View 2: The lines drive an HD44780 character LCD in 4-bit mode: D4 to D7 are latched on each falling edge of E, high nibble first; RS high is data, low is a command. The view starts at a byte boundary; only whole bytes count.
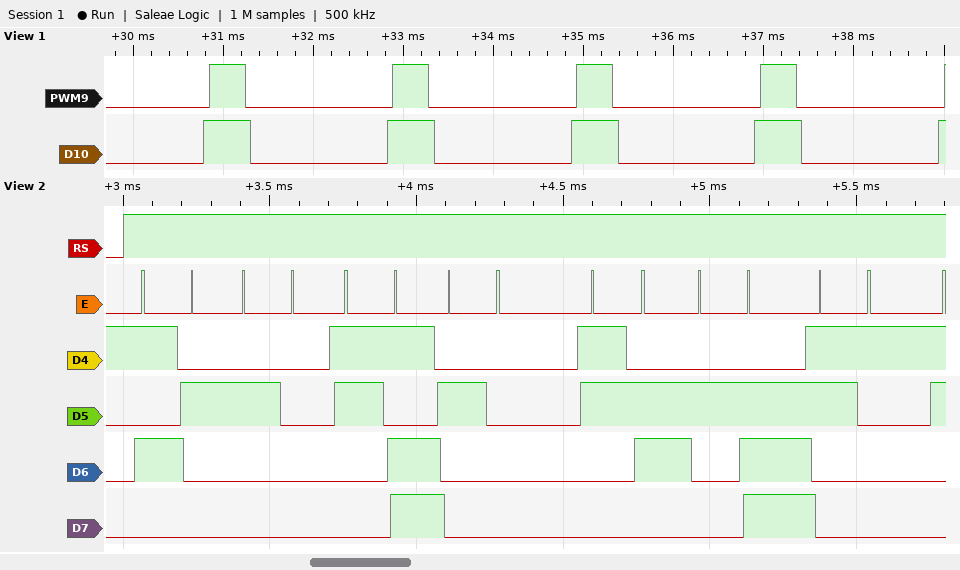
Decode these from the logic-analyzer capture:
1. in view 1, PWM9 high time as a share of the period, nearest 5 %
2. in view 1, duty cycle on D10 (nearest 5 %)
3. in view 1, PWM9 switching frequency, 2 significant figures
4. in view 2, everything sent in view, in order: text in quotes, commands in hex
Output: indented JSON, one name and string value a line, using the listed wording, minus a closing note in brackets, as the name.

{
  "in view 1, PWM9 high time as a share of the period, nearest 5 %": "20 %",
  "in view 1, duty cycle on D10": "25 %",
  "in view 1, PWM9 switching frequency, 2 significant figures": "490 Hz",
  "in view 2, everything sent in view, in order: text in quotes, commands in hex": "\"R = 6.1\""
}
